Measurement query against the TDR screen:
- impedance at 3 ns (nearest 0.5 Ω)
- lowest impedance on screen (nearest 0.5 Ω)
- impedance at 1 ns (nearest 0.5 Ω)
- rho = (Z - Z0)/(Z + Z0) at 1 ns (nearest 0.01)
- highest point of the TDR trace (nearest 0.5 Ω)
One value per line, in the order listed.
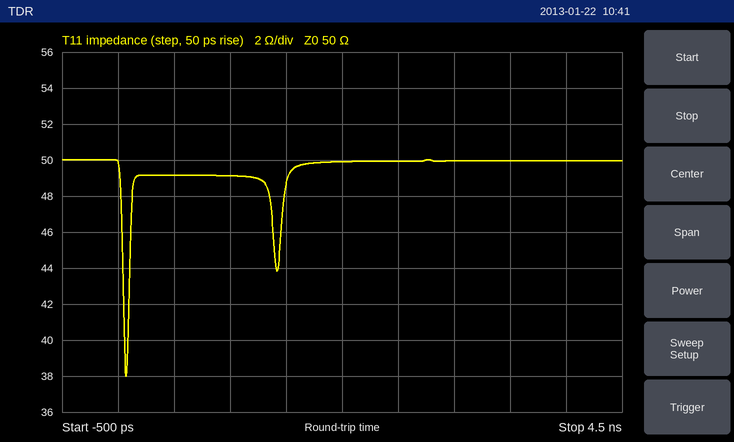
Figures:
50.0 Ω
38.0 Ω
49.0 Ω
-0.01
50.0 Ω
